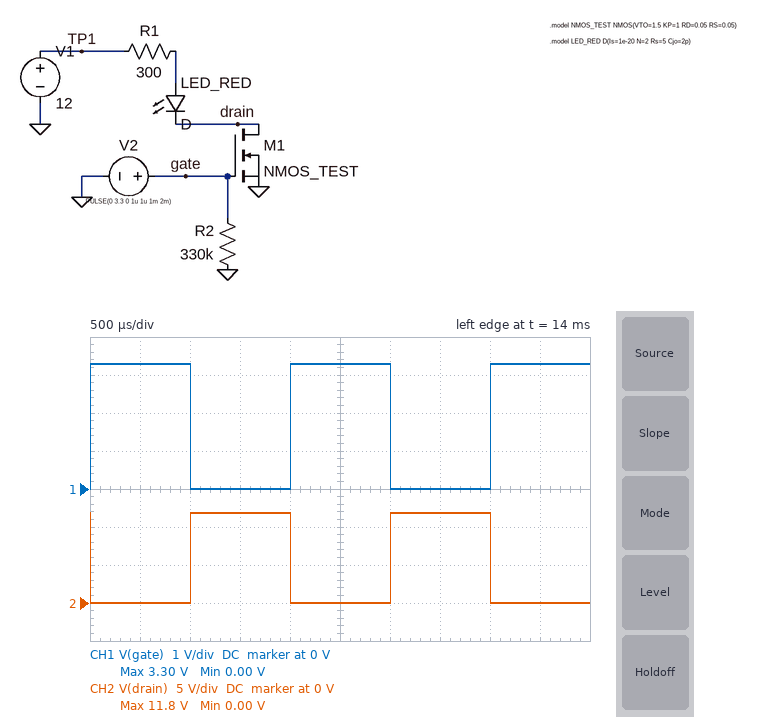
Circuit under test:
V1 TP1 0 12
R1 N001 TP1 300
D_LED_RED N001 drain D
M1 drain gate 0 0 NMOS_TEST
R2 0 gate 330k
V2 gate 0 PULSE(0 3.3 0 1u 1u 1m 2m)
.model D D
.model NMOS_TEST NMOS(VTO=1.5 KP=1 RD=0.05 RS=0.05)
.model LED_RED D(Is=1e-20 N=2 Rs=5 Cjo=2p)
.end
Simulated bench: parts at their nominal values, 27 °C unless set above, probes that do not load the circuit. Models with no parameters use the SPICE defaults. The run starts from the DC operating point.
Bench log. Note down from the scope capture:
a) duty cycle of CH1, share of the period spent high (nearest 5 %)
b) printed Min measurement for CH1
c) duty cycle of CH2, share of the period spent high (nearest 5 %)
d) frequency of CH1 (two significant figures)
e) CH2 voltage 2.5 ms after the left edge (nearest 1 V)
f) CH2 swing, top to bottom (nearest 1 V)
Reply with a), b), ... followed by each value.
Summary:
a) 50 %
b) 0.00 V
c) 50 %
d) 500 Hz
e) 0 V
f) 12 V
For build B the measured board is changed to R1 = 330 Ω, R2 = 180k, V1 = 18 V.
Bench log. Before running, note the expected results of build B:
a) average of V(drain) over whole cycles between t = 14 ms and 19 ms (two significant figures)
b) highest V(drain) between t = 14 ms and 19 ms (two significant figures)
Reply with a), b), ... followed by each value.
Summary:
a) 8.9 V
b) 18 V
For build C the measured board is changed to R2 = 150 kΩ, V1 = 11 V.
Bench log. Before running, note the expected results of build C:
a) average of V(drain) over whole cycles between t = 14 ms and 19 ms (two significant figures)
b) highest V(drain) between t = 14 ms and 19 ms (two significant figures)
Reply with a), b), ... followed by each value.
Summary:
a) 5.4 V
b) 11 V
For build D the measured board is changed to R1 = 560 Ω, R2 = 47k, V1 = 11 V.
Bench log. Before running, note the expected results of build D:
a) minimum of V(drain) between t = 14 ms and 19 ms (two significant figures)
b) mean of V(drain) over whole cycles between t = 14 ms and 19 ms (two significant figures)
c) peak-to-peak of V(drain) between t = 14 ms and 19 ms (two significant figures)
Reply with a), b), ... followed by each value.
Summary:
a) 12 mV
b) 5.4 V
c) 11 V
